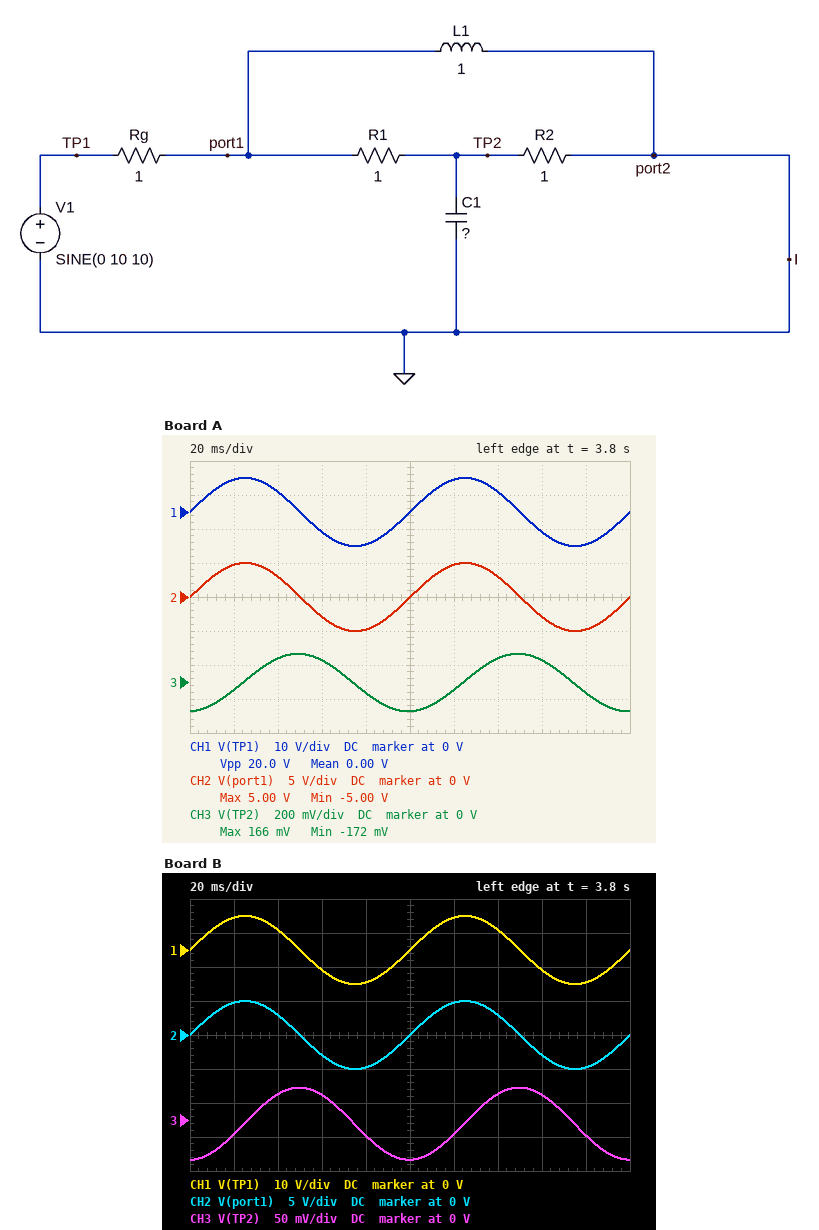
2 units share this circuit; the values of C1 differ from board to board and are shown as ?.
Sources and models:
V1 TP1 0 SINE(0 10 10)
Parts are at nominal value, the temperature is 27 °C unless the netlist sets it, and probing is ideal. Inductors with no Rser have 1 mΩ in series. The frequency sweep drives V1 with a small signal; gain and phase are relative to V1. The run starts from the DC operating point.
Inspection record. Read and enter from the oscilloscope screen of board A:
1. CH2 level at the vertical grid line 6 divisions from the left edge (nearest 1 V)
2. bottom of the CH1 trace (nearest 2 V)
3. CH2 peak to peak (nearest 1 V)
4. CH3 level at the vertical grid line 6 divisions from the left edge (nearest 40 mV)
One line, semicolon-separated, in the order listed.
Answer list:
5 V; -10 V; 10 V; -40 mV
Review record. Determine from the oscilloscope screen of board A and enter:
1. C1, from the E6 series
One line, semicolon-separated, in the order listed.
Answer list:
470 mF
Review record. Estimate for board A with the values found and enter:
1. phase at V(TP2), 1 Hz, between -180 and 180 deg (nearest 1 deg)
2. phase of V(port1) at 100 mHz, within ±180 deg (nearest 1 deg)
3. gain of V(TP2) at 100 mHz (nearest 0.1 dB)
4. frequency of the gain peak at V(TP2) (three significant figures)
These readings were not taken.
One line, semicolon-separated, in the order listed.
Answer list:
-58 deg; 45 deg; -12.7 dB; 232 mHz
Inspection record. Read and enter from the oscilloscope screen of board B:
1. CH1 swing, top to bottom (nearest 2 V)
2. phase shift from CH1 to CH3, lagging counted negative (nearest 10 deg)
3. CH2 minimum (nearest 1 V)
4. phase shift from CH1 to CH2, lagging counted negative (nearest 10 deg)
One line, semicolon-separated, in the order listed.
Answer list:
20 V; -90 deg; -5 V; 0 deg
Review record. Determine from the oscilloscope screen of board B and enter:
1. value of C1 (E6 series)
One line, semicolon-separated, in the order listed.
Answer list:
1.5 F
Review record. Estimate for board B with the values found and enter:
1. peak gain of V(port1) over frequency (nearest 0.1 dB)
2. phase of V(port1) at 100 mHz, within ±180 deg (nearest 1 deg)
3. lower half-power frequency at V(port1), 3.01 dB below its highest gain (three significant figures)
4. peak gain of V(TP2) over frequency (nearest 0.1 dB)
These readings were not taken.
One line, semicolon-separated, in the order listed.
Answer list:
-5.2 dB; 41 deg; 72.3 mHz; -13.1 dB
